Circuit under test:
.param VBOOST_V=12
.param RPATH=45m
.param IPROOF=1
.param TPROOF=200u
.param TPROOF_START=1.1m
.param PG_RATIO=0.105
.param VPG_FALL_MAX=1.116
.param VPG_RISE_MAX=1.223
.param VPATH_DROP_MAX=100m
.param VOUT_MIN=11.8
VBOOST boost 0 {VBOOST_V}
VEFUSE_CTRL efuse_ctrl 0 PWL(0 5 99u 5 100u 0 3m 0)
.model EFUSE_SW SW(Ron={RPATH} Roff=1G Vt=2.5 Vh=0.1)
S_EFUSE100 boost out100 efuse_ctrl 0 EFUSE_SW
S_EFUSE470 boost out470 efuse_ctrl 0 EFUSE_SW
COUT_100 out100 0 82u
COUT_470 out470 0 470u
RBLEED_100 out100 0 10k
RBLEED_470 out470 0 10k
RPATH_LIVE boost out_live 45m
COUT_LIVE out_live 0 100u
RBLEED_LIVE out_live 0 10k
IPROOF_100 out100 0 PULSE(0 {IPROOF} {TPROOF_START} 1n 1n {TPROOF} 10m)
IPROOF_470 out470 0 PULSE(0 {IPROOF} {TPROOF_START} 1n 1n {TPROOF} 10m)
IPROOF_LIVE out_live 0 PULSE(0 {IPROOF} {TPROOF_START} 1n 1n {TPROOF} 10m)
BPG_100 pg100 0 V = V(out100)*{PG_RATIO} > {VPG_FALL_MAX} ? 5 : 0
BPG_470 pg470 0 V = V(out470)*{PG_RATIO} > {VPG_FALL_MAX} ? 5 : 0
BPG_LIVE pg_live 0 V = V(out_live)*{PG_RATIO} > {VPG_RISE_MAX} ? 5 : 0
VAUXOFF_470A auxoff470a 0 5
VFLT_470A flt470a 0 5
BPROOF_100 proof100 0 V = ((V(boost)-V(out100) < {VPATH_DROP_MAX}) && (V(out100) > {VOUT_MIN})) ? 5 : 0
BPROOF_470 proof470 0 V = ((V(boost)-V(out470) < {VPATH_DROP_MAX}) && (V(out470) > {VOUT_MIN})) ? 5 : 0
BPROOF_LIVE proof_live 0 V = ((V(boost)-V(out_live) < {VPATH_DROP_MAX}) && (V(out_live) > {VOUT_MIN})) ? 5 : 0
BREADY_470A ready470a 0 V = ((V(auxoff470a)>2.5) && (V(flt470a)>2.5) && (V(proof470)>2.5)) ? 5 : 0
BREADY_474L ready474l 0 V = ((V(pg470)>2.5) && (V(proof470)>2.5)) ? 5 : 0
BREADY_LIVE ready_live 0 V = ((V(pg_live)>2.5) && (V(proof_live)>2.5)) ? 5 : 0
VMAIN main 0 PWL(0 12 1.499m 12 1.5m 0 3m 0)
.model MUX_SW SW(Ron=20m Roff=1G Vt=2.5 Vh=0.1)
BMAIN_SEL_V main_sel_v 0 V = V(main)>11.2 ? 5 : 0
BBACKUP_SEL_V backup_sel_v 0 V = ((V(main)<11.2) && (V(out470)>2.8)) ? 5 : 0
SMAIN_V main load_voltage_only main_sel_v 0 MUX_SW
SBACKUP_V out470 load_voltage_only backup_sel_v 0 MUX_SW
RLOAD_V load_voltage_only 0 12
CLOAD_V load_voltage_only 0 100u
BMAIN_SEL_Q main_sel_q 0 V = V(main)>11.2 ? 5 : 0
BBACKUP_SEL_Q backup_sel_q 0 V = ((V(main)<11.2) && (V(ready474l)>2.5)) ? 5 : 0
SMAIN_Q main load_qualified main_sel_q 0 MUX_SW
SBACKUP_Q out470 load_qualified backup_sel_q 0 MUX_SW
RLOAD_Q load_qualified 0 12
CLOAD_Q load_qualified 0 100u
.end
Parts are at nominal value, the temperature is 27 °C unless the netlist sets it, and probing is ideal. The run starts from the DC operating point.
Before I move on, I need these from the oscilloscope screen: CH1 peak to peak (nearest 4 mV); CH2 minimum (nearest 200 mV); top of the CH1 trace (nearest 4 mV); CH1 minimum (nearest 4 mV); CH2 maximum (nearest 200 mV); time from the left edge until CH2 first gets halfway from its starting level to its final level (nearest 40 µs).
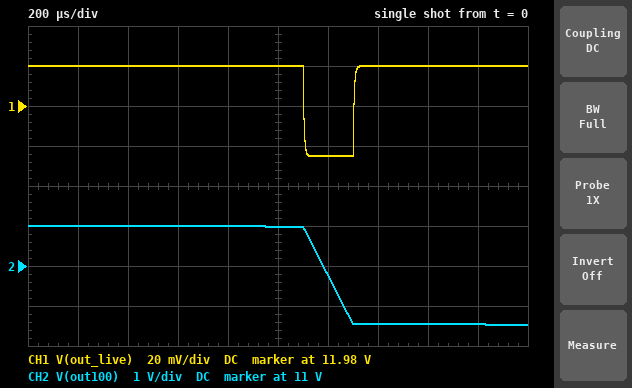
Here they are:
44 mV
9.6 V
12.000 V
11.956 V
12.0 V
1.20 ms
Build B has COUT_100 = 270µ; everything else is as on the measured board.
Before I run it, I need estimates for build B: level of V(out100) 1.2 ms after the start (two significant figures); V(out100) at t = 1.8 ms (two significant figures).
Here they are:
12 V
11 V
